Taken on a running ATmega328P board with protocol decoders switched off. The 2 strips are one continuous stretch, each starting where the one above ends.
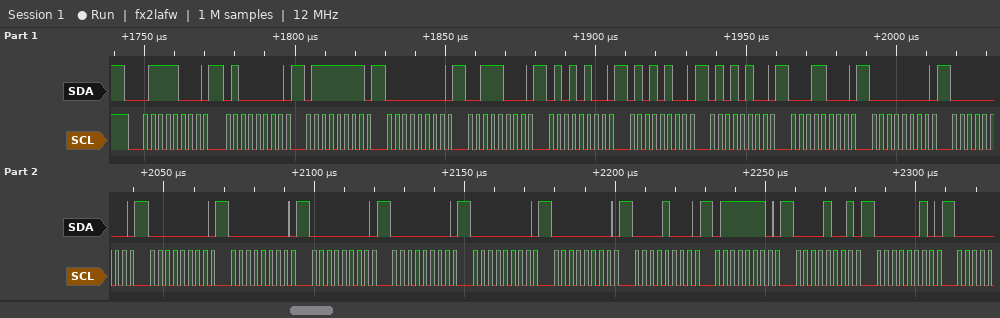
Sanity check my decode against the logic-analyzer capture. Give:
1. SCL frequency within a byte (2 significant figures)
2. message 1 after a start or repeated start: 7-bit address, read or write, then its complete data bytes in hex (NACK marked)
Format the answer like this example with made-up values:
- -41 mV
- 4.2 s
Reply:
- 400 kHz
- 0x3C write: 40 7F 00 38 54 54 54 18 00 00 00 00 00 00 00 00 08 7E 09 02
